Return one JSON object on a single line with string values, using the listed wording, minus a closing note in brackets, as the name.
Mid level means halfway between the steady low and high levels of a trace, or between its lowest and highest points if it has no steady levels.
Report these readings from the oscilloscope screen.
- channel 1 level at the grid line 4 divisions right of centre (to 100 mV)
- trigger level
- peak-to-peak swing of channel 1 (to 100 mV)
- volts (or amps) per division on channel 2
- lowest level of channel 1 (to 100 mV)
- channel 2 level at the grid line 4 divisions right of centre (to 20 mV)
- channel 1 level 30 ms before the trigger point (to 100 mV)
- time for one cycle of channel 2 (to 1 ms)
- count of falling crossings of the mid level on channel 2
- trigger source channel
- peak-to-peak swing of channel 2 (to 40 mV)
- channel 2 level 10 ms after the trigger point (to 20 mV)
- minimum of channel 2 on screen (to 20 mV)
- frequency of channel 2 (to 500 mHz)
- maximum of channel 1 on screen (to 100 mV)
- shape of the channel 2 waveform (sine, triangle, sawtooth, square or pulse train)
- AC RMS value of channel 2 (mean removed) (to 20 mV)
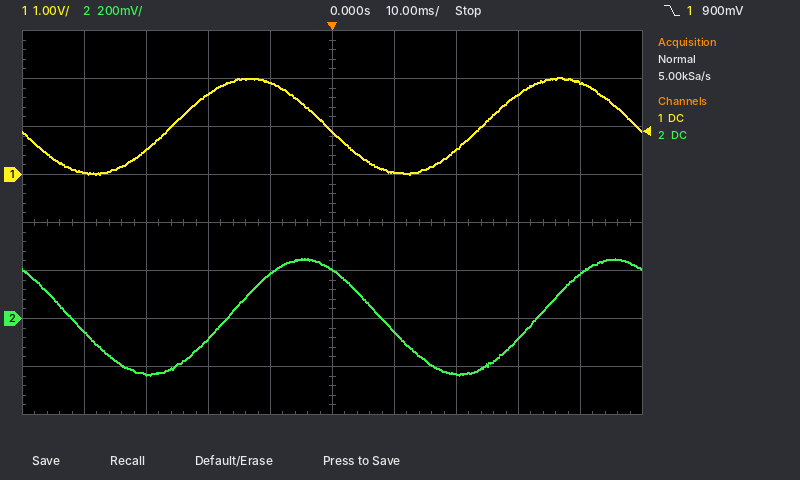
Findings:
{"channel 1 level at the grid line 4 divisions right of centre": "1.9 V", "trigger level": "900 mV", "peak-to-peak swing of channel 1": "2.0 V", "volts (or amps) per division on channel 2": "200 mV", "lowest level of channel 1": "0.0 V", "channel 2 level at the grid line 4 divisions right of centre": "180 mV", "channel 1 level 30 ms before the trigger point": "500 mV", "time for one cycle of channel 2": "50 ms", "count of falling crossings of the mid level on channel 2": "2", "trigger source channel": "channel 1", "peak-to-peak swing of channel 2": "480 mV", "channel 2 level 10 ms after the trigger point": "-60 mV", "minimum of channel 2 on screen": "-240 mV", "frequency of channel 2": "20.0 Hz", "maximum of channel 1 on screen": "2.0 V", "shape of the channel 2 waveform": "sine", "AC RMS value of channel 2 (mean removed)": "160 mV"}
